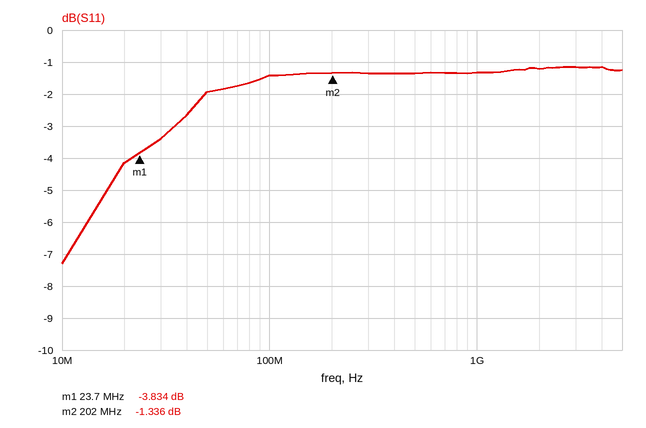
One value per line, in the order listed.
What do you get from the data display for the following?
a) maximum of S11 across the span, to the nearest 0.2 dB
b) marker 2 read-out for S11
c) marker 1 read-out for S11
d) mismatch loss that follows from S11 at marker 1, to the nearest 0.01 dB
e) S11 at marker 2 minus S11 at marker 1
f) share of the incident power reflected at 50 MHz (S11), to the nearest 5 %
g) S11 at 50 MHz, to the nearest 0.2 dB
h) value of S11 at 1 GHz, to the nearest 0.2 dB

-1.2 dB
-1.336 dB
-3.834 dB
2.32 dB
2.498 dB
65 %
-2.0 dB
-1.4 dB
